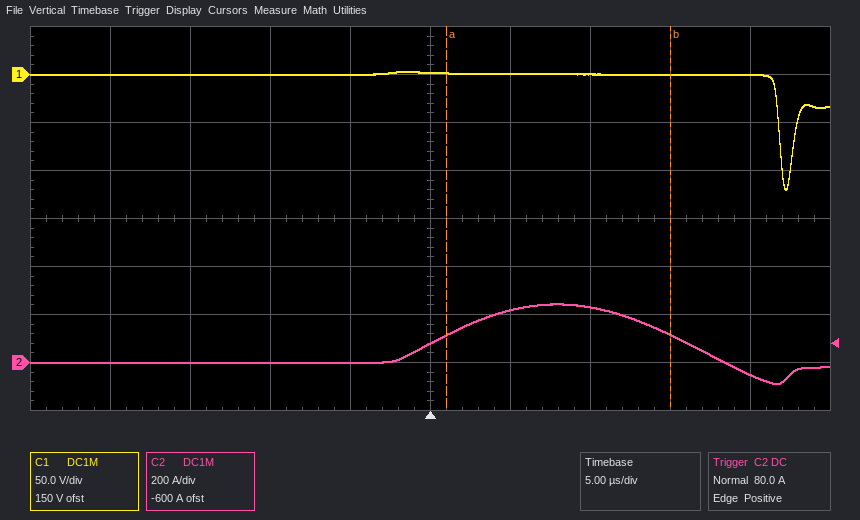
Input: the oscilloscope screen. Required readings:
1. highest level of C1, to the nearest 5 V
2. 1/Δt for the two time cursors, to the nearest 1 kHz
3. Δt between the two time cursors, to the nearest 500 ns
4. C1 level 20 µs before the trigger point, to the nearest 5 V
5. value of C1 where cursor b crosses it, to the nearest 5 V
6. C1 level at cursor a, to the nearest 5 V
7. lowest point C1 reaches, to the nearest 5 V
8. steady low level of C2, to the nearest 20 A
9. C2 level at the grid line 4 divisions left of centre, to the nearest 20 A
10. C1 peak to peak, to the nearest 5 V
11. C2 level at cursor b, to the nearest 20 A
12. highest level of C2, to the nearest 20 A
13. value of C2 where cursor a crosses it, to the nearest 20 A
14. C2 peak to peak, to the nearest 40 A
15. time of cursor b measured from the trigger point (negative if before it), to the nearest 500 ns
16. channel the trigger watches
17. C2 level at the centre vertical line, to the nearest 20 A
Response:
5 V
71 kHz
14.0 µs
0 V
0 V
0 V
-120 V
0 A
0 A
125 V
120 A
240 A
120 A
320 A
+15.0 µs
C2
80 A
